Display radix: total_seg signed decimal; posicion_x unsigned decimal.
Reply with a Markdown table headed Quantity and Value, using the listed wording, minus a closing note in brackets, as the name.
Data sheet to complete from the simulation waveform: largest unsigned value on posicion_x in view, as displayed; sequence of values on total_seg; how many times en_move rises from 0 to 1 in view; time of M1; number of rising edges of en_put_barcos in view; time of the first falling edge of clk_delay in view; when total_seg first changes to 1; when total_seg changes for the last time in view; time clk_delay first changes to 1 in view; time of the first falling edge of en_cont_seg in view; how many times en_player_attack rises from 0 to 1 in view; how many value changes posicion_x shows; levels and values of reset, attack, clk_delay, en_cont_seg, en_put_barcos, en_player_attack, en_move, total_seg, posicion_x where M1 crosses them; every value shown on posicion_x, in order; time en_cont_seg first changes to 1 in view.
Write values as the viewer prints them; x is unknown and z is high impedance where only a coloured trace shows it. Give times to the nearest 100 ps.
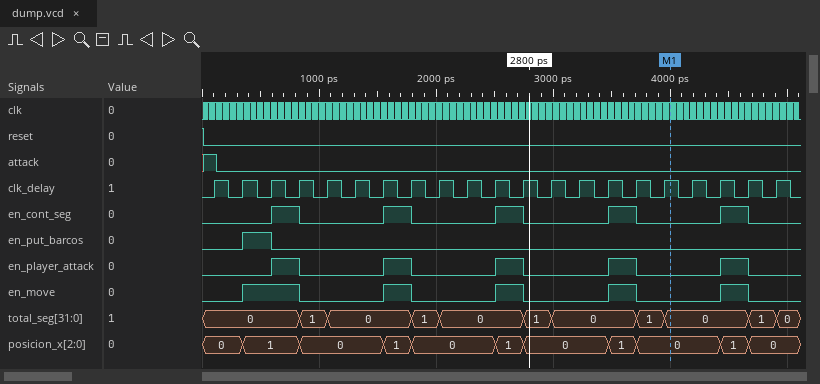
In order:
| Quantity | Value |
|---|---|
| largest unsigned value on posicion_x in view, as displayed | 1 |
| sequence of values on total_seg | 0, 1, 0, 1, 0, 1, 0, 1, 0, 1, 0 |
| how many times en_move rises from 0 to 1 in view | 5 |
| time of M1 | 4000 ps |
| number of rising edges of en_put_barcos in view | 1 |
| time of the first falling edge of clk_delay in view | 200 ps |
| when total_seg first changes to 1 | 800 ps |
| when total_seg changes for the last time in view | 4900 ps |
| time clk_delay first changes to 1 in view | 100 ps |
| time of the first falling edge of en_cont_seg in view | 800 ps |
| how many times en_player_attack rises from 0 to 1 in view | 5 |
| how many value changes posicion_x shows | 10 |
| levels and values of reset, attack, clk_delay, en_cont_seg, en_put_barcos, en_player_attack, en_move, total_seg, posicion_x where M1 crosses them | reset=0, attack=0, clk_delay=1, en_cont_seg=0, en_put_barcos=0, en_player_attack=0, en_move=0, total_seg=0, posicion_x=0 |
| every value shown on posicion_x, in order | 0, 1, 0, 1, 0, 1, 0, 1, 0, 1, 0 |
| time en_cont_seg first changes to 1 in view | 600 ps |
